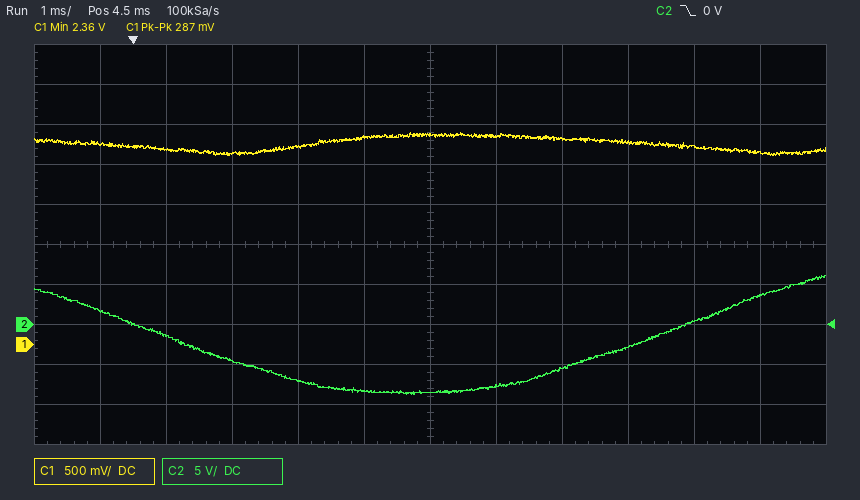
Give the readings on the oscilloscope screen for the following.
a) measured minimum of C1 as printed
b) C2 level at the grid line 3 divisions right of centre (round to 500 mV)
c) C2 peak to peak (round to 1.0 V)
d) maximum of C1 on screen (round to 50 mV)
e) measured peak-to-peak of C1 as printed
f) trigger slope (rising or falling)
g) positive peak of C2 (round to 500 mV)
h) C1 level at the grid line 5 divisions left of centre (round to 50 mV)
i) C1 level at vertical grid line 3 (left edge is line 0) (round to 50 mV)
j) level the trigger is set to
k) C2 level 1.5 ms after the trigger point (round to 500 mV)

2.36 V
-3.0 V
15.0 V
2.65 V
287 mV
falling
6.0 V
2.50 V
2.40 V
0 V
-4.5 V
